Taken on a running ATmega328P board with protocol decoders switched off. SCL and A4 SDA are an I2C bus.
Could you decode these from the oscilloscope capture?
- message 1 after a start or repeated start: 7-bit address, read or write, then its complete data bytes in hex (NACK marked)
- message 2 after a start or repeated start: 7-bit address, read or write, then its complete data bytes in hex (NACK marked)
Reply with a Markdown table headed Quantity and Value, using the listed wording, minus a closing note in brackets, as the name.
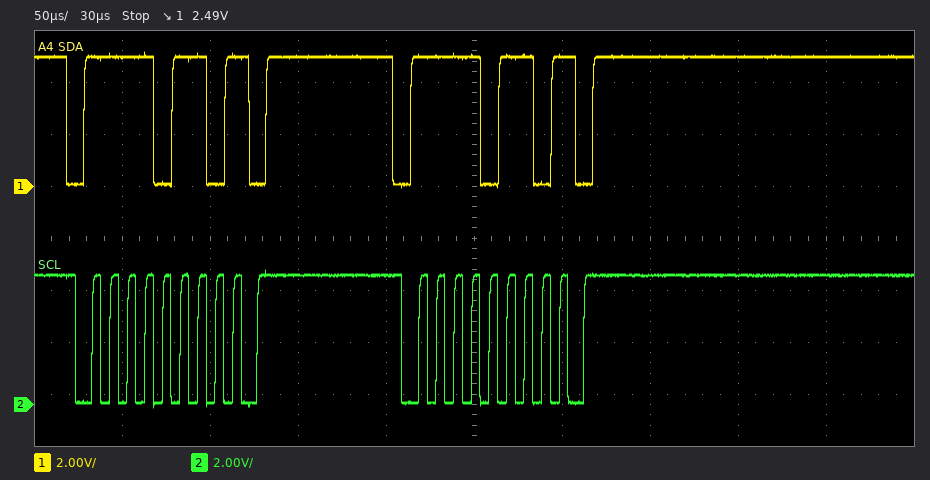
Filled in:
| Quantity | Value |
|---|---|
| message 1 after a start or repeated start: 7-bit address, read or write, then its complete data bytes in hex | 0x7B write NACK |
| message 2 after a start or repeated start: 7-bit address, read or write, then its complete data bytes in hex | 0x7B write NACK |
